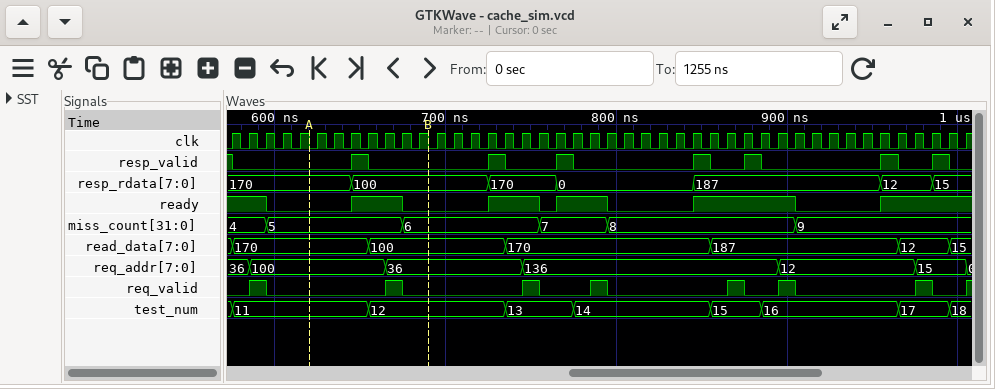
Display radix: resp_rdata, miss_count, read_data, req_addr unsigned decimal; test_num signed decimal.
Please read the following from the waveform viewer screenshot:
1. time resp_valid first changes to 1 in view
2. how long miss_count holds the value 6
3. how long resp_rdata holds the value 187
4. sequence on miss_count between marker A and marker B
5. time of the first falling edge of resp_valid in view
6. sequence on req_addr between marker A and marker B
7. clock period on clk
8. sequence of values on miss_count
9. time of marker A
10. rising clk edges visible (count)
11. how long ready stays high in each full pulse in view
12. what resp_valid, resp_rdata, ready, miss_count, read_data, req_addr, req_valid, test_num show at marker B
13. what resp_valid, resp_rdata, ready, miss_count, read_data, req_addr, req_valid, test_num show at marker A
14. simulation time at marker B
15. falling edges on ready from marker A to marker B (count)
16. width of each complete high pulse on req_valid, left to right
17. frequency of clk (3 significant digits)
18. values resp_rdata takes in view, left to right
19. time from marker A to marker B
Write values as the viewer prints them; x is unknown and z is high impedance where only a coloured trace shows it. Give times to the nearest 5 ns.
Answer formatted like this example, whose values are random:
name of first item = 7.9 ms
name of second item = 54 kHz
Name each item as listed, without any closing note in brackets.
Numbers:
time resp_valid first changes to 1 in view = 645 ns
how long miss_count holds the value 6 = 80 ns
how long resp_rdata holds the value 187 = 110 ns
sequence on miss_count between marker A and marker B = 5, 6
time of the first falling edge of resp_valid in view = 575 ns
sequence on req_addr between marker A and marker B = 100, 36
clock period on clk = 10 ns
sequence of values on miss_count = 4, 5, 6, 7, 8, 9
time of marker A = 620 ns
rising clk edges visible = 44
how long ready stays high in each full pulse in view = 30 ns, 30 ns, 30 ns, 60 ns
what resp_valid, resp_rdata, ready, miss_count, read_data, req_addr, req_valid, test_num show at marker B = resp_valid=0, resp_rdata=100, ready=0, miss_count=6, read_data=100, req_addr=36, req_valid=0, test_num=12
what resp_valid, resp_rdata, ready, miss_count, read_data, req_addr, req_valid, test_num show at marker A = resp_valid=0, resp_rdata=170, ready=0, miss_count=5, read_data=170, req_addr=100, req_valid=0, test_num=11
simulation time at marker B = 690 ns
falling edges on ready from marker A to marker B = 1
width of each complete high pulse on req_valid, left to right = 10 ns, 10 ns, 10 ns, 10 ns, 10 ns, 10 ns, 10 ns
frequency of clk = 100 MHz
values resp_rdata takes in view, left to right = 170, 100, 170, 0, 187, 12, 15
time from marker A to marker B = 70 ns
